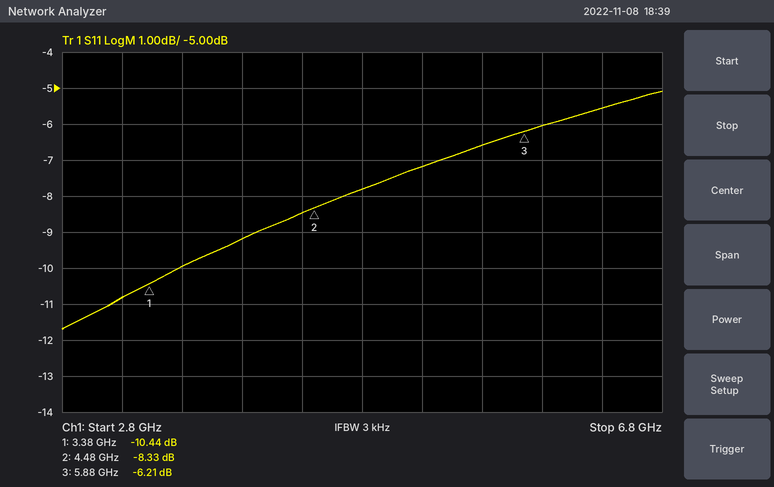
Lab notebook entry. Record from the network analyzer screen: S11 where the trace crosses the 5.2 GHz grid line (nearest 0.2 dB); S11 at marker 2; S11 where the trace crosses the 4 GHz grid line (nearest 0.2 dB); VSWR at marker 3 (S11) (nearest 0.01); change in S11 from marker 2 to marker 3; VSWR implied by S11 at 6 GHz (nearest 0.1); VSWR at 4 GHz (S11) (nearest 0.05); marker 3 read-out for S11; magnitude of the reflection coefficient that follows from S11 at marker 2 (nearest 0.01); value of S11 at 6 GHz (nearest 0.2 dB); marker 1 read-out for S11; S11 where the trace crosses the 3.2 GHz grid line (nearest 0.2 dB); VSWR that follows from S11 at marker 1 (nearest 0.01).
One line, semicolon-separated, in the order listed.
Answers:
-7.2 dB; -8.33 dB; -9.2 dB; 2.92; 2.12 dB; 3.0; 2.05; -6.21 dB; 0.38; -6.0 dB; -10.44 dB; -10.8 dB; 1.86
